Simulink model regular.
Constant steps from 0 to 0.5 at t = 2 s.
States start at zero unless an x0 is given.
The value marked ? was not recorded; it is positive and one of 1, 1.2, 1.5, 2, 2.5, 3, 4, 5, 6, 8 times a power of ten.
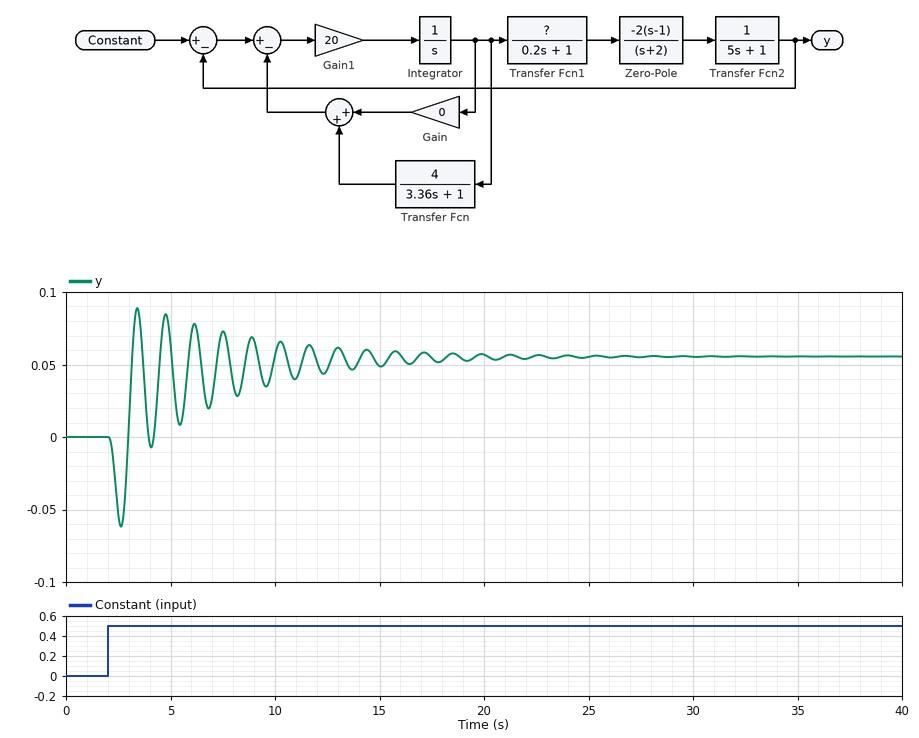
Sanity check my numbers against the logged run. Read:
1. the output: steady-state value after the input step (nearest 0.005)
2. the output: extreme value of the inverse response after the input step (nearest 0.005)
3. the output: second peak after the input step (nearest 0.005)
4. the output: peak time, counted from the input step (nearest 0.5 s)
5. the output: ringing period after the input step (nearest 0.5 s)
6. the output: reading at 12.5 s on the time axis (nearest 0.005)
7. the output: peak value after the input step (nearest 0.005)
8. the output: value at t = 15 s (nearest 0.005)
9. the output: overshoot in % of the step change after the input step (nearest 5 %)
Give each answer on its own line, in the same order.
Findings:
0.055
-0.060
0.085
1.5 s
1.5 s
0.045
0.090
0.050
60 %
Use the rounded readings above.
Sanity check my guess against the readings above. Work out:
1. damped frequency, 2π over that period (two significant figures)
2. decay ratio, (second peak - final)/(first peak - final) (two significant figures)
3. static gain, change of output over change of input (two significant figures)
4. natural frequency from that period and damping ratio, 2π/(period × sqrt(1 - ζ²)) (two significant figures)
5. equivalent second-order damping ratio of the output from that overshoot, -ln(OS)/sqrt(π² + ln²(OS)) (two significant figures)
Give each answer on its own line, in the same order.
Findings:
4.2 rad/s
0.86
0.11
4.2 rad/s
0.16
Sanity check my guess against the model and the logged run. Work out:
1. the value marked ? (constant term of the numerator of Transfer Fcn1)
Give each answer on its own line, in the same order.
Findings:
0.5
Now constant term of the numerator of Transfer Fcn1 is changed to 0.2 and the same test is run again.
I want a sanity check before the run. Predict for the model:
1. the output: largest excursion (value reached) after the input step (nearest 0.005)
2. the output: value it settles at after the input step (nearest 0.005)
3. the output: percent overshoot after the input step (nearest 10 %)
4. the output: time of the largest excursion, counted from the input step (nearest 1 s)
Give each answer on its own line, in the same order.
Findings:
0.035
0.025
40 %
3 s
